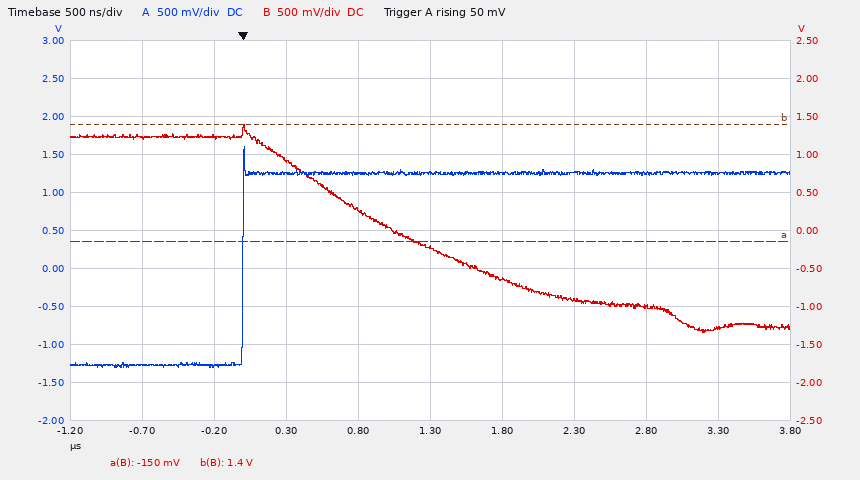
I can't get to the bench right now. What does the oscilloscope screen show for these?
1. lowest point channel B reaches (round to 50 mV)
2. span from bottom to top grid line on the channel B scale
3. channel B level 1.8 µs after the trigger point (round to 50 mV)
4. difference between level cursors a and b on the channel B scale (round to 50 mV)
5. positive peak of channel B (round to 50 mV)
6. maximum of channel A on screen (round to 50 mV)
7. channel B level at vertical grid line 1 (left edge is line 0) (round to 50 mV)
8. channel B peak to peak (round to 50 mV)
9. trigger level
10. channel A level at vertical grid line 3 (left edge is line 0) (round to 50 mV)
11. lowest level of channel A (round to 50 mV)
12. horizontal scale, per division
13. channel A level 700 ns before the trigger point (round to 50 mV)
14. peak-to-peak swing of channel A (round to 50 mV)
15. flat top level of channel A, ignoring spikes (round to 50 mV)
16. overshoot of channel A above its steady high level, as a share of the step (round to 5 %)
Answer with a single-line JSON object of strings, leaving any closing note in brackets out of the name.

{"lowest point channel B reaches": "-1.35 V", "span from bottom to top grid line on the channel B scale": "5 V", "channel B level 1.8 µs after the trigger point": "-650 mV", "difference between level cursors a and b on the channel B scale": "1.55 V", "positive peak of channel B": "1.40 V", "maximum of channel A on screen": "1.60 V", "channel B level at vertical grid line 1 (left edge is line 0)": "1.20 V", "channel B peak to peak": "2.75 V", "trigger level": "50 mV", "channel A level at vertical grid line 3 (left edge is line 0)": "1.25 V", "lowest level of channel A": "-1.30 V", "horizontal scale, per division": "500 ns", "channel A level 700 ns before the trigger point": "-1.25 V", "peak-to-peak swing of channel A": "2.90 V", "flat top level of channel A, ignoring spikes": "1.25 V", "overshoot of channel A above its steady high level, as a share of the step": "15 %"}
